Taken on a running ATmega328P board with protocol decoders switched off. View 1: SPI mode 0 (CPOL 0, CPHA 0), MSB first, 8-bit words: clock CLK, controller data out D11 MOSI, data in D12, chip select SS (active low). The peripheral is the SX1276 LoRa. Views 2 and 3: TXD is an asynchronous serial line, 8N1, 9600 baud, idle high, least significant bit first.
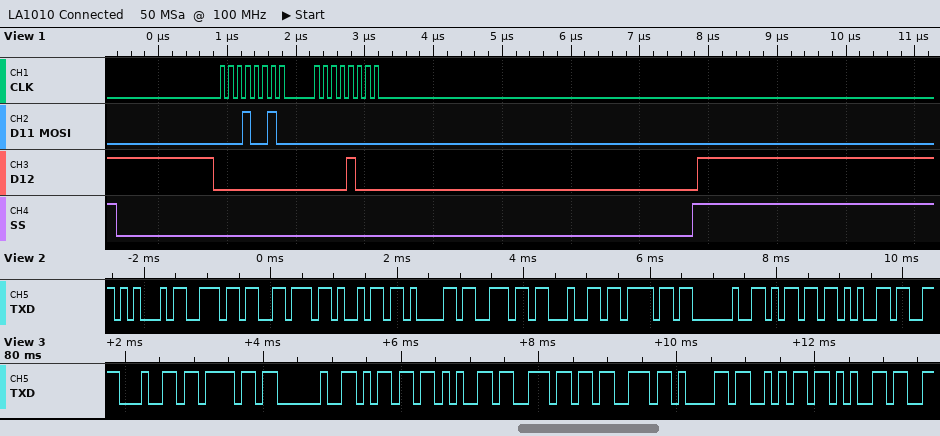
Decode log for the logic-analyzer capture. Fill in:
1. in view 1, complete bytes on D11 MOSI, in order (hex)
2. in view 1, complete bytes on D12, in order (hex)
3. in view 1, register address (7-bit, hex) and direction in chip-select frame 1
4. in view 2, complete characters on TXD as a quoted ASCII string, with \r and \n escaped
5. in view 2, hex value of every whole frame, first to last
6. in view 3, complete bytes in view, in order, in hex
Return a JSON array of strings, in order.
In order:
["0x12 0x00", "0x00 0x08", "0x12 read", "\"Enviando me\"", "0x45 0x6E 0x76 0x69 0x61 0x6E 0x64 0x6F 0x20 0x6D 0x65", "0x64 0x6F 0x20 0x6D 0x65 0x6E 0x73 0x61 0x6A 0x65"]
